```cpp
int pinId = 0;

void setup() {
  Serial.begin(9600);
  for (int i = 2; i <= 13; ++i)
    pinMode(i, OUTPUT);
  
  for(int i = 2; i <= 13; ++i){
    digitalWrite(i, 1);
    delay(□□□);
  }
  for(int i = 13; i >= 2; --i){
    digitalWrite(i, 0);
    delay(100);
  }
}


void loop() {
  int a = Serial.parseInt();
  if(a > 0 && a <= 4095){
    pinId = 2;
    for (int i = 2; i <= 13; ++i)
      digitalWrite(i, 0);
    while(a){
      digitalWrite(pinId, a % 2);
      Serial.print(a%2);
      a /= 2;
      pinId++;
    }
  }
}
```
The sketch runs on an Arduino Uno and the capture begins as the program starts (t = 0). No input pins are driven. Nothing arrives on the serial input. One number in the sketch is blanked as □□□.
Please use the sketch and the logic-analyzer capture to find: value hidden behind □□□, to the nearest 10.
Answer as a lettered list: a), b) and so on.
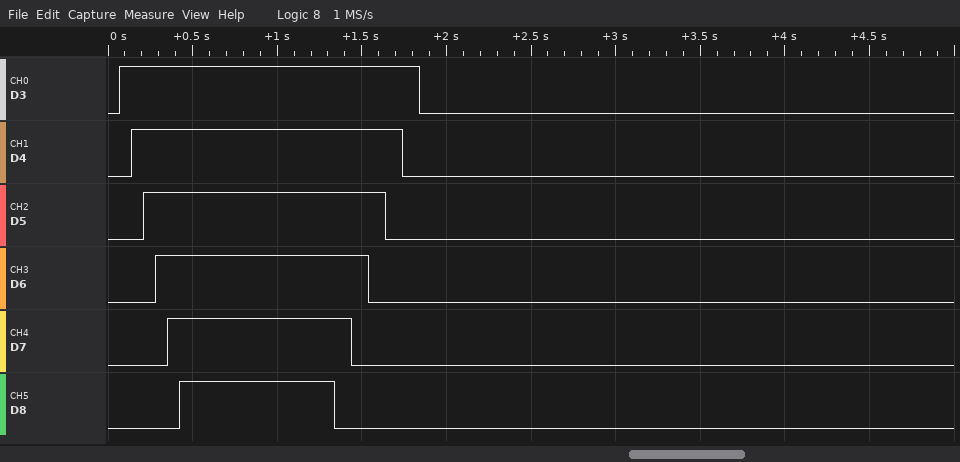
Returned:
a) 70
